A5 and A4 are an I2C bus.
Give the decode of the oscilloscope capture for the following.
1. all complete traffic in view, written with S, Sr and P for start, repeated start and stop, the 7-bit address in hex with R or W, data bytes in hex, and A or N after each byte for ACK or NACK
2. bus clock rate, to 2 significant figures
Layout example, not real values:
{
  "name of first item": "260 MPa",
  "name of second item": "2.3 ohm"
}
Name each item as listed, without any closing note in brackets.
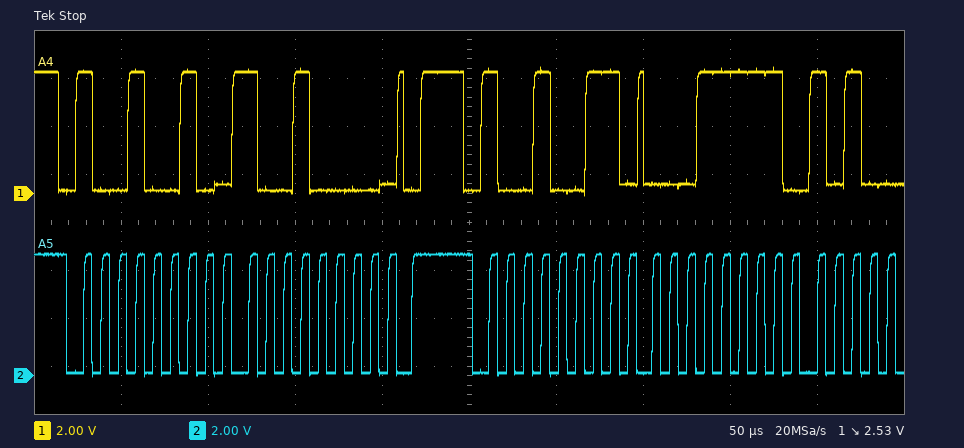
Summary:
{
  "all complete traffic in view, written with S, Sr and P for start, repeated start and stop, the 7-bit address in hex with R or W, data bytes in hex, and A or N after each byte for ACK or NACK": "S 49W A 90 A P S 49R A 1F A",
  "bus clock rate, to 2 significant figures": "100 kHz"
}
